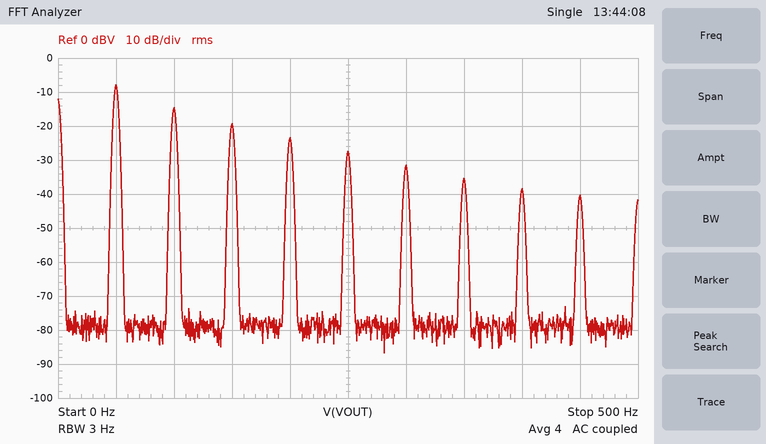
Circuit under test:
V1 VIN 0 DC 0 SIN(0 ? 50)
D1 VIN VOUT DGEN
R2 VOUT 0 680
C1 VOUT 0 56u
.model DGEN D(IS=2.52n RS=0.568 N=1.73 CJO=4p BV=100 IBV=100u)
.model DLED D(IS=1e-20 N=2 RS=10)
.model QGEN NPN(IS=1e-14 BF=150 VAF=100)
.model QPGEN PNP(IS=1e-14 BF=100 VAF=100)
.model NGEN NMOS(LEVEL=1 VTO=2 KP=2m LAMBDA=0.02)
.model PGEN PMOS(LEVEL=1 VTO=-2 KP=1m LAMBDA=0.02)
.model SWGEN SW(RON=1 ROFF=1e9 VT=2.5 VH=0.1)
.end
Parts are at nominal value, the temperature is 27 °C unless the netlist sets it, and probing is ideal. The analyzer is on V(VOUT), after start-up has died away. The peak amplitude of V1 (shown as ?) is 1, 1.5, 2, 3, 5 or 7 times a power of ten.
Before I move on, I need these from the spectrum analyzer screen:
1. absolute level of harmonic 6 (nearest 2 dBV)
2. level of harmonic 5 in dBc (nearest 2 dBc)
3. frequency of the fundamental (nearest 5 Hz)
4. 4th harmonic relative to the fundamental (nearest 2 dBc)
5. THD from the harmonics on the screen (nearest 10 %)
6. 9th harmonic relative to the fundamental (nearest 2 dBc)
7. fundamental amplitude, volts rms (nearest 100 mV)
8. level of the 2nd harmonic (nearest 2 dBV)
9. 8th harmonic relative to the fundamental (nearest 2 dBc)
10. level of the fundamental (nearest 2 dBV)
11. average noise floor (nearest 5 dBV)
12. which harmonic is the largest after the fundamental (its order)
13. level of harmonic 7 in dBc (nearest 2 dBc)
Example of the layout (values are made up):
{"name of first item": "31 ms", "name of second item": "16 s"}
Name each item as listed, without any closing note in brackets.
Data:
{"absolute level of harmonic 6": "-32 dBV", "level of harmonic 5 in dBc": "-20 dBc", "frequency of the fundamental": "50 Hz", "4th harmonic relative to the fundamental": "-16 dBc", "THD from the harmonics on the screen": "60 %", "9th harmonic relative to the fundamental": "-32 dBc", "fundamental amplitude, volts rms": "400 mV", "level of the 2nd harmonic": "-14 dBV", "8th harmonic relative to the fundamental": "-30 dBc", "level of the fundamental": "-8 dBV", "average noise floor": "-80 dBV", "which harmonic is the largest after the fundamental": "2", "level of harmonic 7 in dBc": "-28 dBc"}
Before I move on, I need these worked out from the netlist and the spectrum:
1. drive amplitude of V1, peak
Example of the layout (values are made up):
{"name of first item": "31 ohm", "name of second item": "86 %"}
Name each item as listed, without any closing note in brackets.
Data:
{"drive amplitude of V1, peak": "5 V"}
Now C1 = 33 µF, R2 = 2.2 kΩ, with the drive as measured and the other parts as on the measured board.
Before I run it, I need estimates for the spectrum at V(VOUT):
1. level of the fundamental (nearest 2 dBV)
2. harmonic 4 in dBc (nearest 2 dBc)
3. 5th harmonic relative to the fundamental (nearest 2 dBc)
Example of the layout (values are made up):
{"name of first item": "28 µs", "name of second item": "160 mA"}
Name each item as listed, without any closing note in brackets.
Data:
{"level of the fundamental": "-12 dBV", "harmonic 4 in dBc": "-14 dBc", "5th harmonic relative to the fundamental": "-18 dBc"}
